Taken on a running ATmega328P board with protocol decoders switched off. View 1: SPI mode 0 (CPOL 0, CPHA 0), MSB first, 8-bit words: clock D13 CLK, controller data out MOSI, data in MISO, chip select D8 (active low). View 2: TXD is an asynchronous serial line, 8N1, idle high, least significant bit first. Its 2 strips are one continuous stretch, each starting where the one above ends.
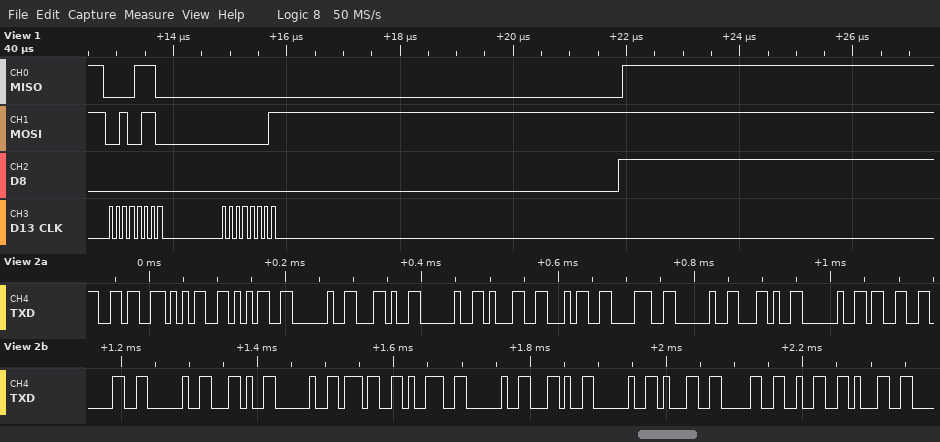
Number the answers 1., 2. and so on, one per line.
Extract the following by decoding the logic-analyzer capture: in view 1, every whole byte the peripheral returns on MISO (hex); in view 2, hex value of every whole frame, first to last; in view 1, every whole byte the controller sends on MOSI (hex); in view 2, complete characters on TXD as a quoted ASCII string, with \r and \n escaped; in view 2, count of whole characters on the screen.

1. 0x0E 0x00
2. 36 35 35 20 2C 20 31 34 38 20 2C 20 33 30 20 2C 20 37 39 20 2C 20 31 30 32 31
3. 0x26 0x01
4. "655 , 148 , 30 , 79 , 1021"
5. 26
